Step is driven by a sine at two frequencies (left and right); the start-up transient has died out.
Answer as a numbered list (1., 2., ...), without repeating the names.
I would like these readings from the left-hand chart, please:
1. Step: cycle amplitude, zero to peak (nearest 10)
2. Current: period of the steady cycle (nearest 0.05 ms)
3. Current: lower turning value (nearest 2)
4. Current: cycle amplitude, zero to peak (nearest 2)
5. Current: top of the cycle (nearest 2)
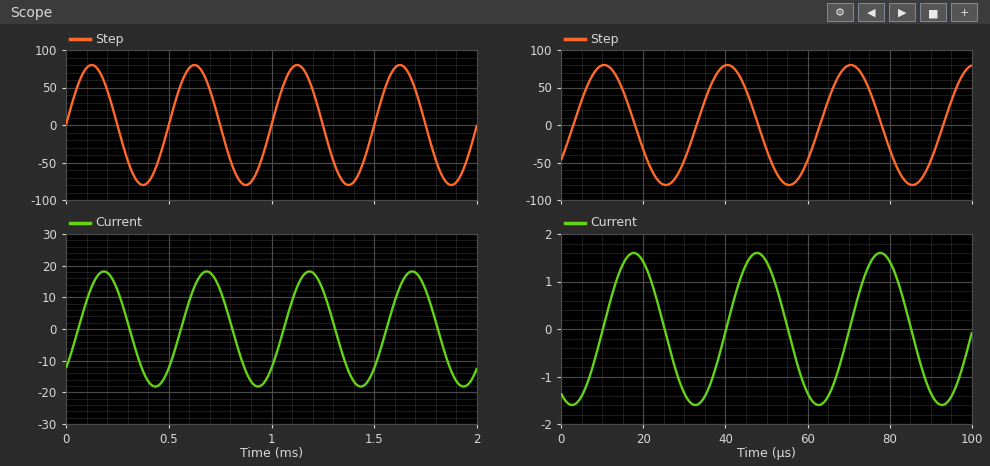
1. 80
2. 0.50 ms
3. -18
4. 18
5. 18
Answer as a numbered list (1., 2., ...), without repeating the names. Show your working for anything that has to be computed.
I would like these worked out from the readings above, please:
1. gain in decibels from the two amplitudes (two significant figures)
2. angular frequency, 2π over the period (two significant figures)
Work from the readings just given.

1. 20 log10(18 / 80) = -13 dB
2. 2π / 0.5 = 13 rad/ms
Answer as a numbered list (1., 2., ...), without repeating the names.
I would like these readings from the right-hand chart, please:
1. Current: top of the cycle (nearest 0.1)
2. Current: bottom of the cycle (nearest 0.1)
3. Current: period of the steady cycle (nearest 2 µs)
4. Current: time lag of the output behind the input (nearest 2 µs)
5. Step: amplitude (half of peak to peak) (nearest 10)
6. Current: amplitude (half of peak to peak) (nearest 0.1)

1. 1.6
2. -1.6
3. 30 µs
4. 8 µs
5. 80
6. 1.6
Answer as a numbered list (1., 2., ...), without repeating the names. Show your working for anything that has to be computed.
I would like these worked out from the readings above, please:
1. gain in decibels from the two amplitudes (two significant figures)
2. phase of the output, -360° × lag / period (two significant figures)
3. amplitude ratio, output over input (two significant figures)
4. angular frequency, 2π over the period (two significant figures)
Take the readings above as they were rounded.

1. 20 log10(1.6 / 80) = -34 dB
2. -360 × 8 / 30 = -96°
3. 1.6 / 80 = 0.020
4. 2π / 30 = 0.21 rad/µs
